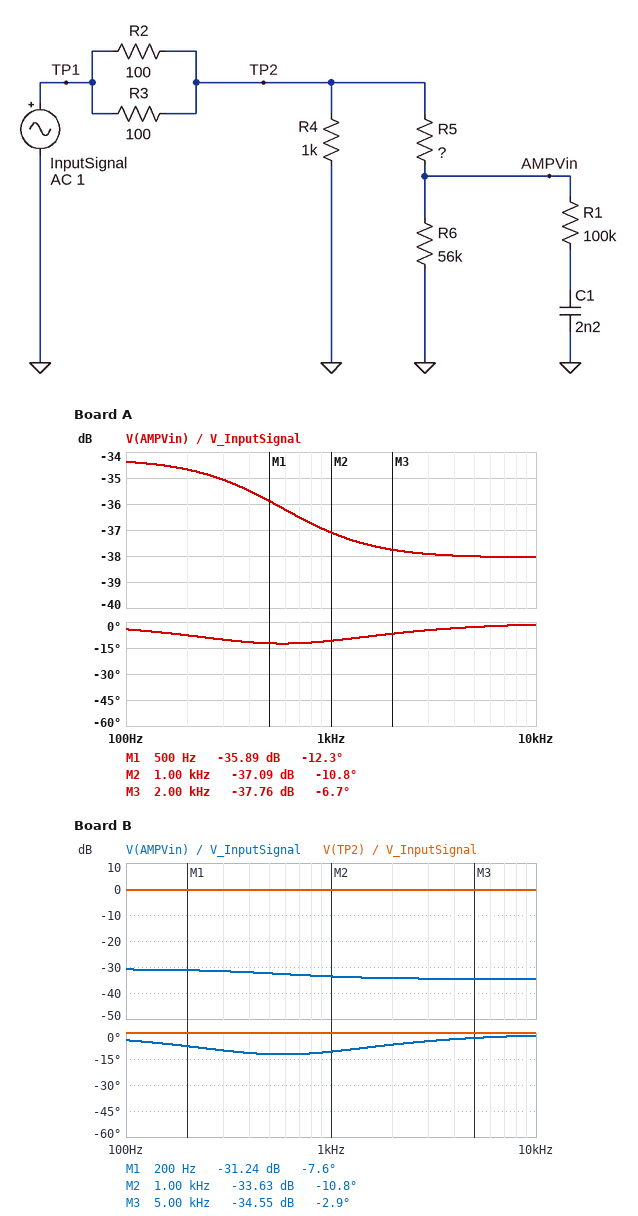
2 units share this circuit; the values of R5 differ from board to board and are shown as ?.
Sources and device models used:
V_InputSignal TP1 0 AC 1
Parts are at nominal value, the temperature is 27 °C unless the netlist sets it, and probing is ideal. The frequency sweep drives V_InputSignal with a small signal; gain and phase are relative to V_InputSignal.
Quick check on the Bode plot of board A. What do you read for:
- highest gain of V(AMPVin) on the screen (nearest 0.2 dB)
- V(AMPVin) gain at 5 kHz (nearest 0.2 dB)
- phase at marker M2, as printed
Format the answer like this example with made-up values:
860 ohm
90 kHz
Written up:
-34.4 dB
-38.0 dB
-10.8 deg
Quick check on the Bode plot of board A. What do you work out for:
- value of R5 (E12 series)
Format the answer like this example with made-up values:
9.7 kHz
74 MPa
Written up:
2.7 MΩ
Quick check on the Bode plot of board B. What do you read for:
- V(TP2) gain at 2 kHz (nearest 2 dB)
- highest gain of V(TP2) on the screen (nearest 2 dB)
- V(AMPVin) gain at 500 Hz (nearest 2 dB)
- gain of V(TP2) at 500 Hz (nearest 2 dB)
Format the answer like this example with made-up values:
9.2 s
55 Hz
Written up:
0 dB
0 dB
-32 dB
0 dB
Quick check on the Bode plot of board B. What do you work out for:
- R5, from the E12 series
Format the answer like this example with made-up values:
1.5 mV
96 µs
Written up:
1.8 MΩ
